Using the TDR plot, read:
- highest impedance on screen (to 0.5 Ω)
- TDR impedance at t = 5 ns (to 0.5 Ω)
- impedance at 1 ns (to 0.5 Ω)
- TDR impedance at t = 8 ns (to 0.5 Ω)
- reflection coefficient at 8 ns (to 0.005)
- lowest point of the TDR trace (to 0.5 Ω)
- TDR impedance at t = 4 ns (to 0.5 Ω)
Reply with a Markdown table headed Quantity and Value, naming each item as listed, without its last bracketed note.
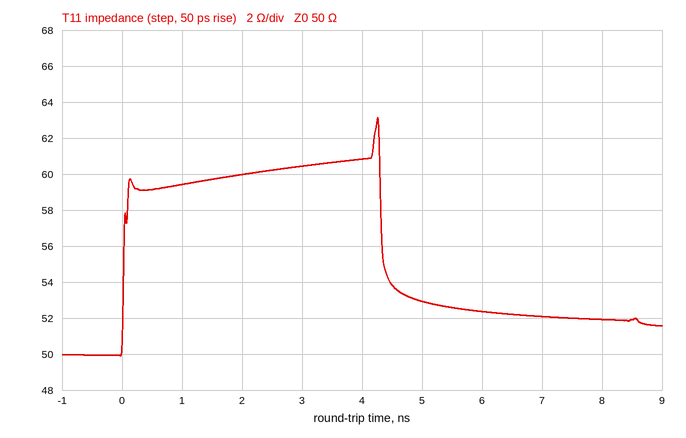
| Quantity | Value |
|---|---|
| highest impedance on screen | 63.0 Ω |
| TDR impedance at t = 5 ns | 53.0 Ω |
| impedance at 1 ns | 59.5 Ω |
| TDR impedance at t = 8 ns | 52.0 Ω |
| reflection coefficient at 8 ns | +0.020 |
| lowest point of the TDR trace | 50.0 Ω |
| TDR impedance at t = 4 ns | 61.0 Ω |
